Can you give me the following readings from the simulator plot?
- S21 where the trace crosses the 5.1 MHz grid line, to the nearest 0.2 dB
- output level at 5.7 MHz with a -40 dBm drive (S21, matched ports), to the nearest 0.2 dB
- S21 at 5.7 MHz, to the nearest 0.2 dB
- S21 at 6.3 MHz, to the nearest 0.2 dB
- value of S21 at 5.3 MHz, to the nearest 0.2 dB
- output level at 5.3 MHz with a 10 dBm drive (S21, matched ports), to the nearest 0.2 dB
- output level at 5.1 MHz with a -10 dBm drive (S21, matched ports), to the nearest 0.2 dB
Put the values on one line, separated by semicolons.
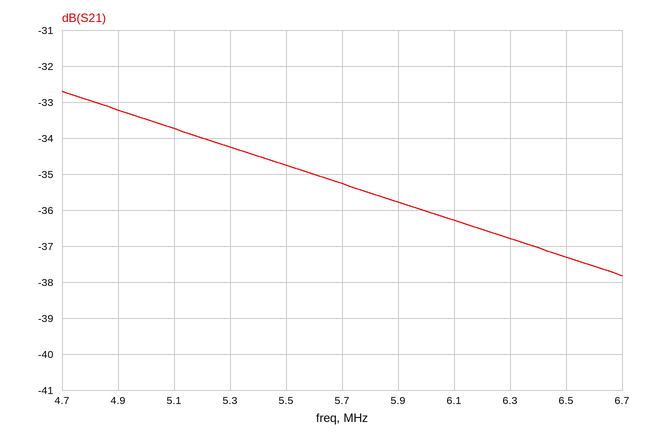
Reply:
-33.8 dB; -75.2 dBm; -35.2 dB; -36.8 dB; -34.2 dB; -24.2 dBm; -43.8 dBm
